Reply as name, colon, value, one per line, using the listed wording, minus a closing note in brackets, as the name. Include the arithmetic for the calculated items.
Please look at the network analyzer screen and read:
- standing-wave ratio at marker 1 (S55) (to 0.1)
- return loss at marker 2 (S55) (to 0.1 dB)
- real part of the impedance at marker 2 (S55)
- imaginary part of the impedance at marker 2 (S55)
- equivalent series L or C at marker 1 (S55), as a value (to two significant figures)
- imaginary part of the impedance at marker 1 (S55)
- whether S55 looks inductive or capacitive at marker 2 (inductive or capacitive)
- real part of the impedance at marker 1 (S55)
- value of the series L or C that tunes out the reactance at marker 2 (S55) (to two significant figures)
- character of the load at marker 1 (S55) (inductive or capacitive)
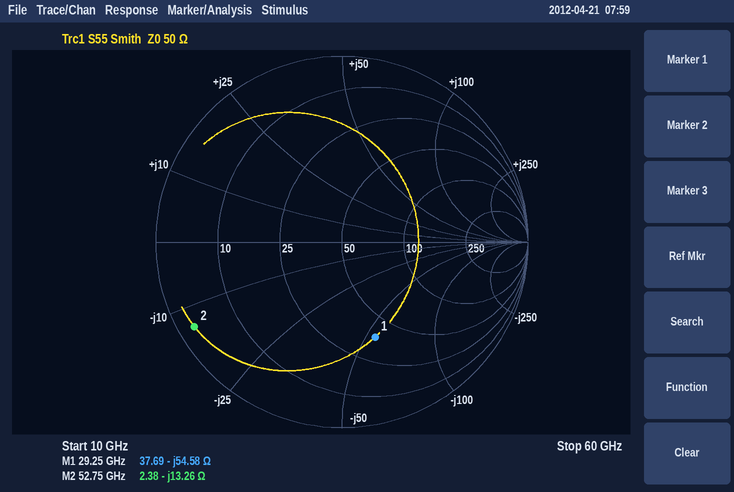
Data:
standing-wave ratio at marker 1 (S55): 3.4
return loss at marker 2 (S55): 0.8 dB
real part of the impedance at marker 2: 2.38 Ω
imaginary part of the impedance at marker 2: -13.26 Ω
equivalent series L or C at marker 1 (S55), as a value: C = 1/(2π × 29.25 GHz × 54.58 Ω) ≈ 100 fF
imaginary part of the impedance at marker 1: -54.58 Ω
whether S55 looks inductive or capacitive at marker 2: capacitive
real part of the impedance at marker 1: 37.69 Ω
value of the series L or C that tunes out the reactance at marker 2 (S55): L = 13.26 Ω/(2π × 52.75 GHz) ≈ 40 pH
character of the load at marker 1 (S55): capacitive
